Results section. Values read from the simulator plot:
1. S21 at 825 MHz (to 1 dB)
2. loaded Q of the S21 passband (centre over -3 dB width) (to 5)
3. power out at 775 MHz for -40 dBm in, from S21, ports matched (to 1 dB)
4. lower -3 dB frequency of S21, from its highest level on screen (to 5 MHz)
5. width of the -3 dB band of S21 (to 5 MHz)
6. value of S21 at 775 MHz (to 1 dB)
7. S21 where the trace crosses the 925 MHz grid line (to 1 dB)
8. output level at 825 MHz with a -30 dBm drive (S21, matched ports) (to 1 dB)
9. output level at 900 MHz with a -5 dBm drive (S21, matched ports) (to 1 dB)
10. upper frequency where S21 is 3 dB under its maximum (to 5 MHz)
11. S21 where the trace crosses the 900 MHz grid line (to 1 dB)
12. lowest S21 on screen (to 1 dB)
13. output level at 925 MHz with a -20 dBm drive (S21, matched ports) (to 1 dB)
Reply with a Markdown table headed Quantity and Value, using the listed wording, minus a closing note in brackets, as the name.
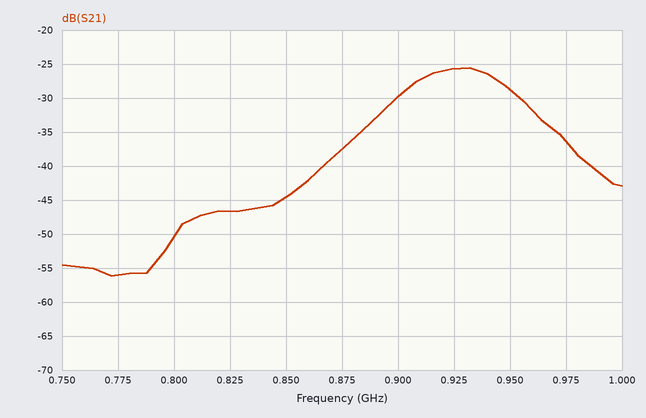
| Quantity | Value |
|---|---|
| S21 at 825 MHz | -47 dB |
| loaded Q of the S21 passband (centre over -3 dB width) | 20 |
| power out at 775 MHz for -40 dBm in, from S21, ports matched | -96 dBm |
| lower -3 dB frequency of S21, from its highest level on screen | 905 MHz |
| width of the -3 dB band of S21 | 45 MHz |
| value of S21 at 775 MHz | -56 dB |
| S21 where the trace crosses the 925 MHz grid line | -26 dB |
| output level at 825 MHz with a -30 dBm drive (S21, matched ports) | -77 dBm |
| output level at 900 MHz with a -5 dBm drive (S21, matched ports) | -35 dBm |
| upper frequency where S21 is 3 dB under its maximum | 950 MHz |
| S21 where the trace crosses the 900 MHz grid line | -30 dB |
| lowest S21 on screen | -56 dB |
| output level at 925 MHz with a -20 dBm drive (S21, matched ports) | -46 dBm |
